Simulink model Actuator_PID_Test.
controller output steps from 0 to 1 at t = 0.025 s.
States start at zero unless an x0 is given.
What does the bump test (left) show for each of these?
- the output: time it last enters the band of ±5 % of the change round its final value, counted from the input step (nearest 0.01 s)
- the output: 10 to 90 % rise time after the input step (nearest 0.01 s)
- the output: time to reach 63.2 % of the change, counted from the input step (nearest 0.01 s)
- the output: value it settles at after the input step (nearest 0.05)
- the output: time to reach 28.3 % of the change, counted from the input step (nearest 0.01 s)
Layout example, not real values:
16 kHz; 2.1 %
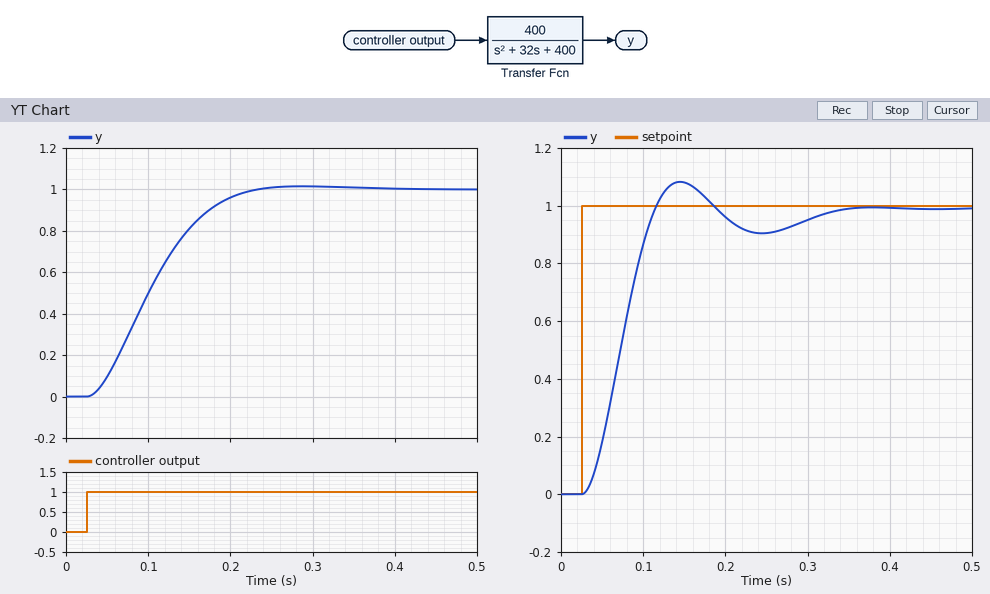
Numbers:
0.17 s; 0.12 s; 0.09 s; 1.00; 0.05 s
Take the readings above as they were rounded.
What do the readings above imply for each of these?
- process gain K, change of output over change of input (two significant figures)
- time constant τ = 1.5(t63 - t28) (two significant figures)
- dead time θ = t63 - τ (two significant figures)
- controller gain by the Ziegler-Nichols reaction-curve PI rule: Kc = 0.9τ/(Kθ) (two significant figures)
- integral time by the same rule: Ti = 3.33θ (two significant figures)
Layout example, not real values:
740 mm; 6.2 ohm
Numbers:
1.0; 0.060 s; 0.030 s; 1.8; 0.100 s
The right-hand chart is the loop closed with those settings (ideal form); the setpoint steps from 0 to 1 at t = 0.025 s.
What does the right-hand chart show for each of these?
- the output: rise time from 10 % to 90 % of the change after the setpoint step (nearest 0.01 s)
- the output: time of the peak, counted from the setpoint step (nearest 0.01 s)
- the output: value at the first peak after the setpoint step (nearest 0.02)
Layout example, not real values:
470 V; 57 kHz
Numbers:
0.06 s; 0.12 s; 1.08
